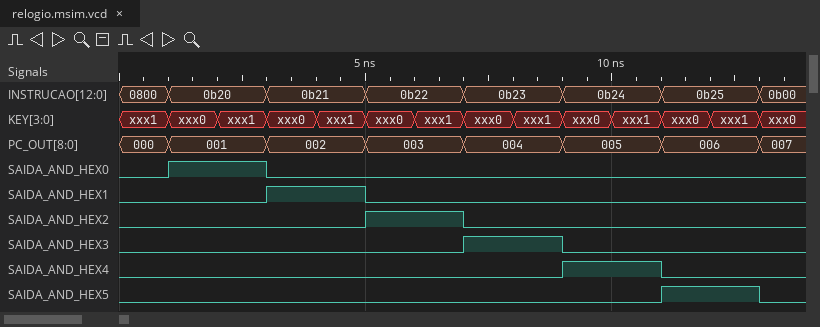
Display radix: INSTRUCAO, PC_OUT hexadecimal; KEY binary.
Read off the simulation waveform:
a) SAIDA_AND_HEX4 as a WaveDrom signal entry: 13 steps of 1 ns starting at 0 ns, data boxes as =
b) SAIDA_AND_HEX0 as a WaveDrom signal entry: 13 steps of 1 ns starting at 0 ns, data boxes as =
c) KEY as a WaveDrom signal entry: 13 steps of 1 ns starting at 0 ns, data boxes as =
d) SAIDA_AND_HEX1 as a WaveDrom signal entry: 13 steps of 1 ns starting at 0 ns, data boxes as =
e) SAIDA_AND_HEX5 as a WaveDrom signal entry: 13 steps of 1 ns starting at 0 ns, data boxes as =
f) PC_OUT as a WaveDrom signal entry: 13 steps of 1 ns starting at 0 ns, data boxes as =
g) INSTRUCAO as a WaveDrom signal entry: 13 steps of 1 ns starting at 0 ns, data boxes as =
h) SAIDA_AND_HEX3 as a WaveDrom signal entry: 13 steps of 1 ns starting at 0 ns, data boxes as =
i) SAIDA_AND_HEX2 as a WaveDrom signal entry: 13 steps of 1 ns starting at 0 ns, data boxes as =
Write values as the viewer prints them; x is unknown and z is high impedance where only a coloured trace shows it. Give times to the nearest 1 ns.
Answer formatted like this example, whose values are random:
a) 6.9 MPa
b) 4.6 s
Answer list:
a) {name: 'SAIDA_AND_HEX4', wave: '0........1.0.'}
b) {name: 'SAIDA_AND_HEX0', wave: '01.0.........'}
c) {name: 'KEY', wave: '=============', data: 'xxx1 xxx0 xxx1 xxx0 xxx1 xxx0 xxx1 xxx0 xxx1 xxx0 xxx1 xxx0 xxx1'}
d) {name: 'SAIDA_AND_HEX1', wave: '0..1.0.......'}
e) {name: 'SAIDA_AND_HEX5', wave: '0..........1.'}
f) {name: 'PC_OUT', wave: '==.=.=.=.=.=.', data: '000 001 002 003 004 005 006'}
g) {name: 'INSTRUCAO', wave: '==.=.=.=.=.=.', data: '0800 0b20 0b21 0b22 0b23 0b24 0b25'}
h) {name: 'SAIDA_AND_HEX3', wave: '0......1.0...'}
i) {name: 'SAIDA_AND_HEX2', wave: '0....1.0.....'}
